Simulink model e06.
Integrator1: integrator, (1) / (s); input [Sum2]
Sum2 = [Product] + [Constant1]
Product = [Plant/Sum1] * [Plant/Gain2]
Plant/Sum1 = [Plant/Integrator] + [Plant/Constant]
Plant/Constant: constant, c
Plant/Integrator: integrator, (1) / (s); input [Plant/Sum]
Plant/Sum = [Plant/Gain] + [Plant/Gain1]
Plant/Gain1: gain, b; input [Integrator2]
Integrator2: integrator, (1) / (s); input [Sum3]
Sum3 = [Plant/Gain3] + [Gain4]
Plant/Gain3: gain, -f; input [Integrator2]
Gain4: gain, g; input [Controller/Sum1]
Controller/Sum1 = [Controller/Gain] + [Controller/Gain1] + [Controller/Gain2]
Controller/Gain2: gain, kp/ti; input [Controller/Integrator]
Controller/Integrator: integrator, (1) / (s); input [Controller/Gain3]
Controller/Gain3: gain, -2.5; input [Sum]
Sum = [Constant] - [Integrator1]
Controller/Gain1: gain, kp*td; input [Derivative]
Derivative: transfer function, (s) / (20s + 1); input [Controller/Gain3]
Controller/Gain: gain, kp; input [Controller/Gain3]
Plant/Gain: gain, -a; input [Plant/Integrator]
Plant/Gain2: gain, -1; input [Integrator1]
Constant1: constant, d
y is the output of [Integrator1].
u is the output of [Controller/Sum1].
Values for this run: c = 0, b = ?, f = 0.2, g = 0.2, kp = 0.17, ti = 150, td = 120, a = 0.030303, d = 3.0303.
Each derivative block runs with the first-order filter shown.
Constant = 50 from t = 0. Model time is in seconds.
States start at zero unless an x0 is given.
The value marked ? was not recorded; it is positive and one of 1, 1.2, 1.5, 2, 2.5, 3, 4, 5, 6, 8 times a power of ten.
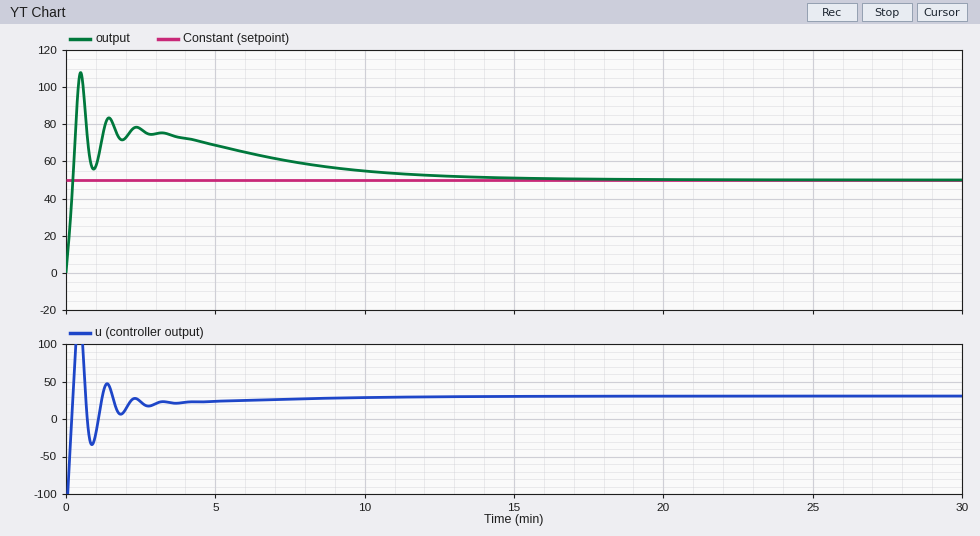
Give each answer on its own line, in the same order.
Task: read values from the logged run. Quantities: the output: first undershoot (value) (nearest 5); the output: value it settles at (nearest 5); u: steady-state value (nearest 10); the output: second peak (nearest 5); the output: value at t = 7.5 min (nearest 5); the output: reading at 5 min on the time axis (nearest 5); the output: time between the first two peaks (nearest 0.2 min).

55
50
30
85
60
70
1.0 min
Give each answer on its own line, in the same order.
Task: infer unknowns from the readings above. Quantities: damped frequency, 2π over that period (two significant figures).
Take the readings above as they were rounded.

6.3 rad/min
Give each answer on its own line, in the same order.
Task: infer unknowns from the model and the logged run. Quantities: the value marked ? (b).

6e-05
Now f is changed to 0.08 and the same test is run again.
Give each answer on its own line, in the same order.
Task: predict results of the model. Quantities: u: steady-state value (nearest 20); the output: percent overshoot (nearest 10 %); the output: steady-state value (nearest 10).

20
170 %
50
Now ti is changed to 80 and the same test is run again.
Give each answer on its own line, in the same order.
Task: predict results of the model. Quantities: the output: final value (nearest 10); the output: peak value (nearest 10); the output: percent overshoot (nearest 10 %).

50
110
120 %
